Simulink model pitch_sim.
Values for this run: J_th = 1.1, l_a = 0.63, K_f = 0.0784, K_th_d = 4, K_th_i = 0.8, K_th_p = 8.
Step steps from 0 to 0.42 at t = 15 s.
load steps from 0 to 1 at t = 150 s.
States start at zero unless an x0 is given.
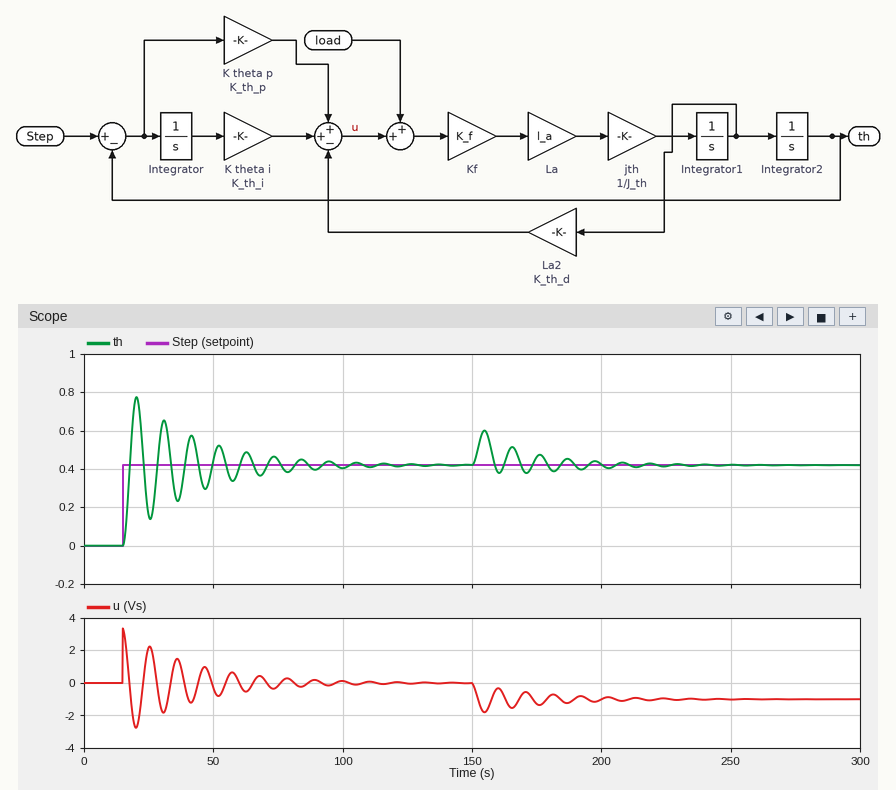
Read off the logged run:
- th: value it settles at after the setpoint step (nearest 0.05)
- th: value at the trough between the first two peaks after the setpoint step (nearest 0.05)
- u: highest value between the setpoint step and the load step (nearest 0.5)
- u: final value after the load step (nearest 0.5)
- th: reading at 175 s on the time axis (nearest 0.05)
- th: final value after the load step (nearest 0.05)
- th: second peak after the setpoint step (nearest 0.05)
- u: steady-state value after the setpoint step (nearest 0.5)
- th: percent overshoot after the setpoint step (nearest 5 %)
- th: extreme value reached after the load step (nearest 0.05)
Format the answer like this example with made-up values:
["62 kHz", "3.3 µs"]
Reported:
["0.40", "0.15", "3.5", "-1.0", "0.45", "0.40", "0.65", "0.0", "85 %", "0.60"]
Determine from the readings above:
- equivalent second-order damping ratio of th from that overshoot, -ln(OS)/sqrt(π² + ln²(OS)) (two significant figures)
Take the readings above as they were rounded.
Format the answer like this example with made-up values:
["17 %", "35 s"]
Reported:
["0.052"]
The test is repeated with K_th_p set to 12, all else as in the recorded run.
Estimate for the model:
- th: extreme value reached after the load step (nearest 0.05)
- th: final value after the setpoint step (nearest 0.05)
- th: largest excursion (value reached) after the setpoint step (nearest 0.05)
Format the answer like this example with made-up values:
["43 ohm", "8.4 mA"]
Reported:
["0.55", "0.40", "0.75"]
